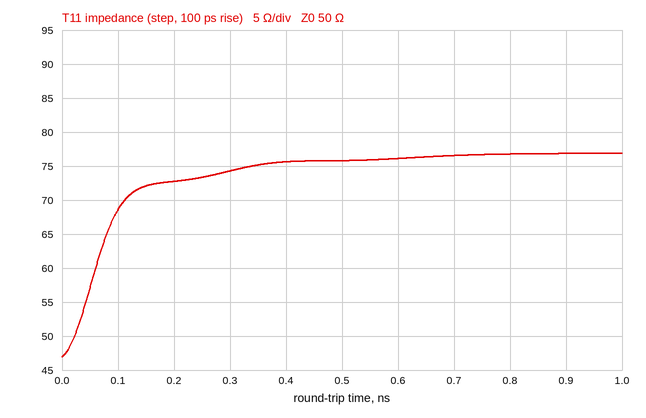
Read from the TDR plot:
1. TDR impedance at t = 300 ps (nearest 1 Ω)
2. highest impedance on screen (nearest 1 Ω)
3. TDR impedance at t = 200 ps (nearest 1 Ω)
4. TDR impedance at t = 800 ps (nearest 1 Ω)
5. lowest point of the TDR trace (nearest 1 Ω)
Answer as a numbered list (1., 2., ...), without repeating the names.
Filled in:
1. 74 Ω
2. 77 Ω
3. 73 Ω
4. 77 Ω
5. 47 Ω
